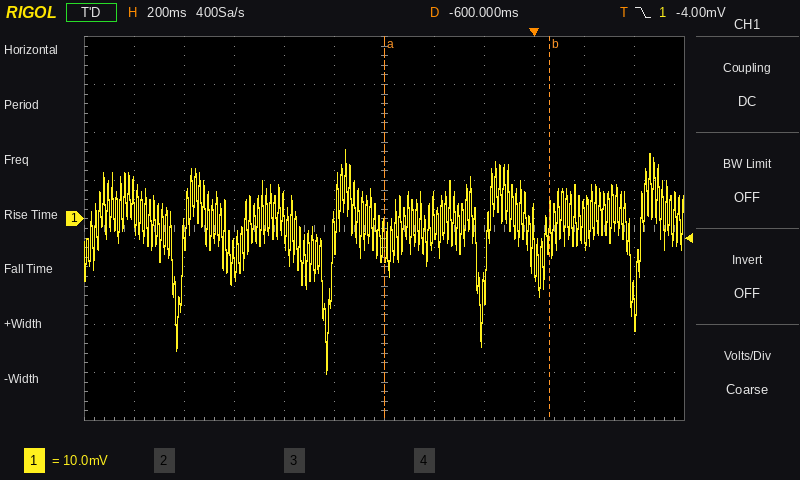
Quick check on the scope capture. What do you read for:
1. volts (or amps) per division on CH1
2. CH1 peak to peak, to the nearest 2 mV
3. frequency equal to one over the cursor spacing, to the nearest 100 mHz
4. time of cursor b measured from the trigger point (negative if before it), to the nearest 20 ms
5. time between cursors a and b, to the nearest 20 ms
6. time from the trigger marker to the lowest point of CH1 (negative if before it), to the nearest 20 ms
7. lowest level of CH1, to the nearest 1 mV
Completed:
10 mV
46 mV
1.5 Hz
+60 ms
660 ms
-820 ms
-32 mV
